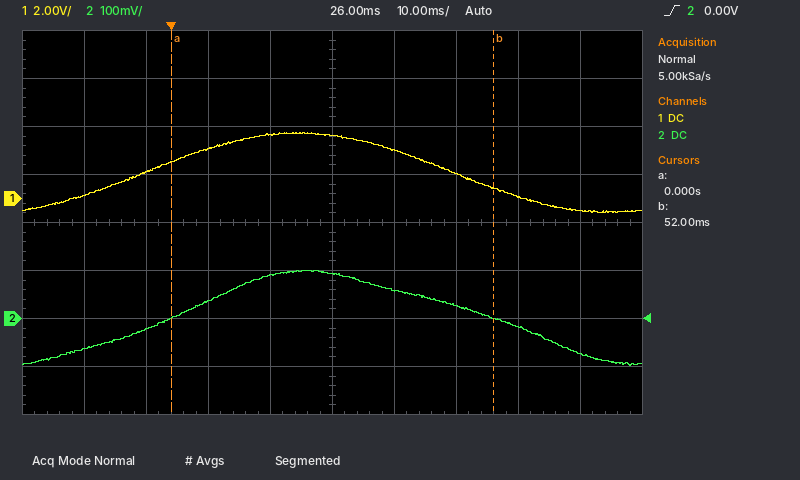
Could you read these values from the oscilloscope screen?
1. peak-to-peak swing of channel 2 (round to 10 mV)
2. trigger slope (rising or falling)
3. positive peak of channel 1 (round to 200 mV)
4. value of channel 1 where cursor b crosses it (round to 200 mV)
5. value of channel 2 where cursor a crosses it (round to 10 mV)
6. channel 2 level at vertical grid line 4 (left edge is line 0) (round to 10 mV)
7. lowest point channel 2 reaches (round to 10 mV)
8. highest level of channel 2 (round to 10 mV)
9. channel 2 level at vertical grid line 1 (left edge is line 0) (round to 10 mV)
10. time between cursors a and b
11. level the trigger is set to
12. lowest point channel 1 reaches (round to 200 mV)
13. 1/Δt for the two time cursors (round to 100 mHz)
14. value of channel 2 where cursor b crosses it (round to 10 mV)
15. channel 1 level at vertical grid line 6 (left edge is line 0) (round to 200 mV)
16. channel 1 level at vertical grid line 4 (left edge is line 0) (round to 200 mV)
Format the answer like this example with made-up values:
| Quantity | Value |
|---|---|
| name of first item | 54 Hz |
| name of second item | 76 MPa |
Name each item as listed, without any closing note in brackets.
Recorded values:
| Quantity | Value |
|---|---|
| peak-to-peak swing of channel 2 | 200 mV |
| trigger slope | rising |
| positive peak of channel 1 | 2.8 V |
| value of channel 1 where cursor b crosses it | 400 mV |
| value of channel 2 where cursor a crosses it | 0 mV |
| channel 2 level at vertical grid line 4 (left edge is line 0) | 90 mV |
| lowest point channel 2 reaches | -100 mV |
| highest level of channel 2 | 100 mV |
| channel 2 level at vertical grid line 1 (left edge is line 0) | -60 mV |
| time between cursors a and b | 52 ms |
| level the trigger is set to | 0.00 V |
| lowest point channel 1 reaches | -600 mV |
| 1/Δt for the two time cursors | 19.2 Hz |
| value of channel 2 where cursor b crosses it | 0 mV |
| channel 1 level at vertical grid line 6 (left edge is line 0) | 2.0 V |
| channel 1 level at vertical grid line 4 (left edge is line 0) | 2.6 V |
